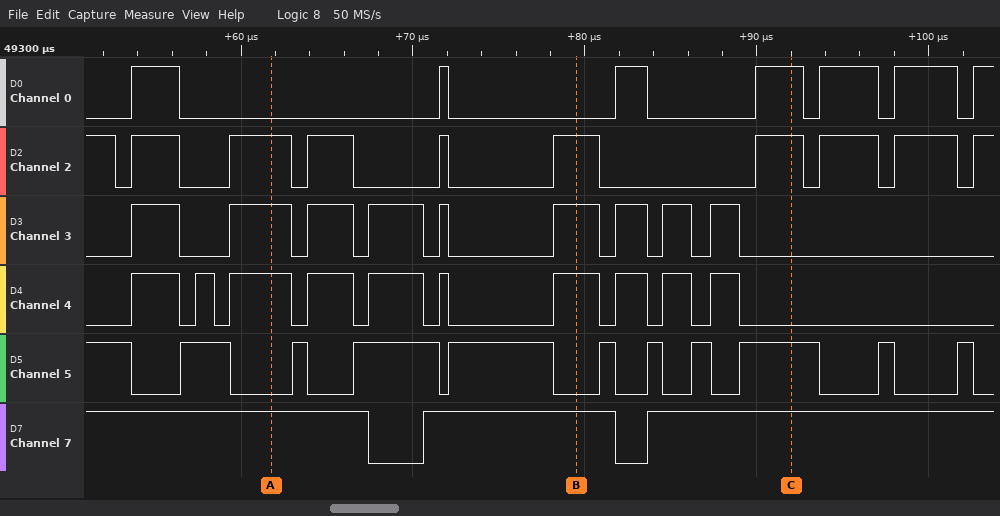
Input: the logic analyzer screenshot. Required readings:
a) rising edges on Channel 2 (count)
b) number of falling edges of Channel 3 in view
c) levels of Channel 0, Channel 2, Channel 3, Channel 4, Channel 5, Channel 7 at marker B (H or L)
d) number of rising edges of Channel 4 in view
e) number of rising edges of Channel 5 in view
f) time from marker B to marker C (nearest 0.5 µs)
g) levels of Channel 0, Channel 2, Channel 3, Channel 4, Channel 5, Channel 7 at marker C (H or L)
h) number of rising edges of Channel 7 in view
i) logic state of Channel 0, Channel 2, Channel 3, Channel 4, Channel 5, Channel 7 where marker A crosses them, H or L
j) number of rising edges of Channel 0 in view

9
9
Channel 0=L, Channel 2=H, Channel 3=H, Channel 4=H, Channel 5=L, Channel 7=H
10
10
12.5 µs
Channel 0=H, Channel 2=H, Channel 3=L, Channel 4=L, Channel 5=H, Channel 7=H
2
Channel 0=L, Channel 2=H, Channel 3=H, Channel 4=H, Channel 5=L, Channel 7=H
7
